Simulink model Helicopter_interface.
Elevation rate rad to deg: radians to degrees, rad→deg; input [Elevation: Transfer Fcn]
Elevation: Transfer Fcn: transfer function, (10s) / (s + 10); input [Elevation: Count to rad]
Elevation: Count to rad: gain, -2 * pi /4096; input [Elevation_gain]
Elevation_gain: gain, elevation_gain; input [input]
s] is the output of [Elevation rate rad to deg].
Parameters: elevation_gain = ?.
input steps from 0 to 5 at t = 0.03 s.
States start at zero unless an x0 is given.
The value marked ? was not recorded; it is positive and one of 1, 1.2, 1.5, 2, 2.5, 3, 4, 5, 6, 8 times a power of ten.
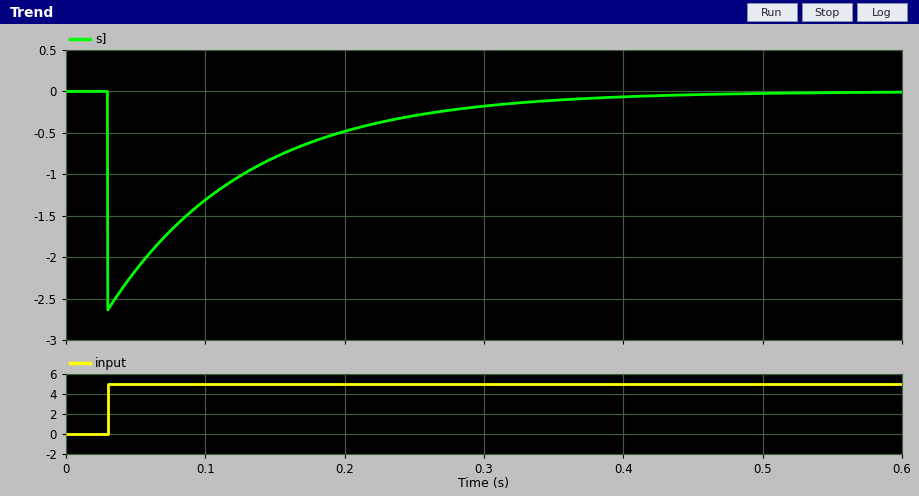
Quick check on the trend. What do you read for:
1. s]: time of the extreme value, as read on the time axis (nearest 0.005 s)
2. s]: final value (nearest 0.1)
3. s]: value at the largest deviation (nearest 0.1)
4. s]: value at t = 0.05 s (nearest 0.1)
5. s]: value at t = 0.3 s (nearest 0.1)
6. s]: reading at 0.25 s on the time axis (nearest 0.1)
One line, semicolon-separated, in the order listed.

0.030 s; 0.0; -2.6; -2.2; -0.2; -0.3
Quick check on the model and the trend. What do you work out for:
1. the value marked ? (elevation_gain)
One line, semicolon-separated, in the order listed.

0.6
